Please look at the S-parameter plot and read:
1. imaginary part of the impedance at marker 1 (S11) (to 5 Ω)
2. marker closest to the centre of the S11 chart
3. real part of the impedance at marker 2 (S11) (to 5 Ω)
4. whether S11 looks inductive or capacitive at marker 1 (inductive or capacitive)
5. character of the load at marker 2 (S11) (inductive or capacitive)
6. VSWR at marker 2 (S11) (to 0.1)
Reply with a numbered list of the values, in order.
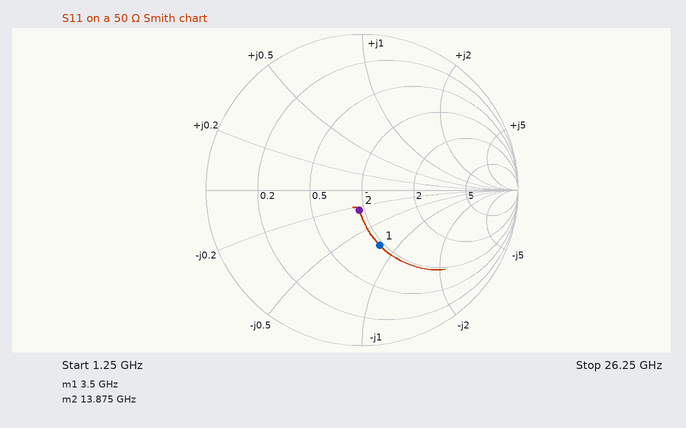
1. -40 Ω
2. marker 2
3. 45 Ω
4. capacitive
5. capacitive
6. 1.3
